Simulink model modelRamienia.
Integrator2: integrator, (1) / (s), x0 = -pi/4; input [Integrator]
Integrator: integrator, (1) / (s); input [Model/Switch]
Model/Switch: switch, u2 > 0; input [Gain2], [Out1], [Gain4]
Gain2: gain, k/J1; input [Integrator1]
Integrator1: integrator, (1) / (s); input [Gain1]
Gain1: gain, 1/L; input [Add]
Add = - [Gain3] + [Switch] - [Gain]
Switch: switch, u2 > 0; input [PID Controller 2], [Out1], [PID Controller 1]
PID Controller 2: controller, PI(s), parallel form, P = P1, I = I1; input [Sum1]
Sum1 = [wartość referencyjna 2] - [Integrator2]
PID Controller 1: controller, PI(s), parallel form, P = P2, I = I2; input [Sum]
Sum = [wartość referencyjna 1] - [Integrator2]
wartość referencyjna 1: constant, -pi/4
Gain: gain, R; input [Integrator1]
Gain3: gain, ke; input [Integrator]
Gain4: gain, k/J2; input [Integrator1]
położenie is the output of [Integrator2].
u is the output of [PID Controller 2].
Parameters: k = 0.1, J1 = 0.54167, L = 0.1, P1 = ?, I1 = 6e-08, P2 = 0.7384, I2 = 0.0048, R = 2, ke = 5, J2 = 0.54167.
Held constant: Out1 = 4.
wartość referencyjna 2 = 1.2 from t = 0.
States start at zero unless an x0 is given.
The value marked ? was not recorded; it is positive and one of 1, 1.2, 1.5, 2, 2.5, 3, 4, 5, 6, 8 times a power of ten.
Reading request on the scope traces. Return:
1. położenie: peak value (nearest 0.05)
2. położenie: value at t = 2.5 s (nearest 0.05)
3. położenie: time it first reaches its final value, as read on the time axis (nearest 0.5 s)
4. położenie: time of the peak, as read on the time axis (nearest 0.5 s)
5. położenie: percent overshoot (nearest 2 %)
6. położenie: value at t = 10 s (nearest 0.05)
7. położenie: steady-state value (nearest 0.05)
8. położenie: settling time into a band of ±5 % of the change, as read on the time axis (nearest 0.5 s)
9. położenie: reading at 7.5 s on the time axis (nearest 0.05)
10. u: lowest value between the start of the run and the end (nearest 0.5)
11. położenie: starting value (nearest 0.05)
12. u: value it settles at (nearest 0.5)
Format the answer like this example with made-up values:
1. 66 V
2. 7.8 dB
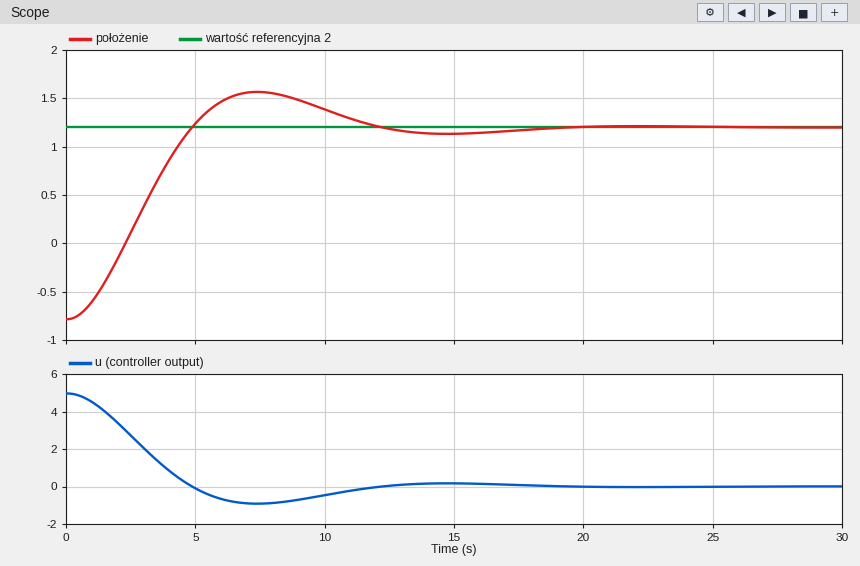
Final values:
1. 1.55
2. 0.10
3. 5.0 s
4. 7.5 s
5. 18 %
6. 1.40
7. 1.20
8. 11.0 s
9. 1.55
10. -1.0
11. -0.80
12. 0.0
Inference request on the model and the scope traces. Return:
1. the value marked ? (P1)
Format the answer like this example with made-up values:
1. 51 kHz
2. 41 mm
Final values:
1. 2.5
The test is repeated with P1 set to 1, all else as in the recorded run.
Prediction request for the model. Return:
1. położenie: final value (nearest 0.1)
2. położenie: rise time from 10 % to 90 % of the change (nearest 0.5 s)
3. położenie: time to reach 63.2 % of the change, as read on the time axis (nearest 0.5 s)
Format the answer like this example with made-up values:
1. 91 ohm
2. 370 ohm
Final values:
1. 1.2
2. 7.5 s
3. 6.0 s
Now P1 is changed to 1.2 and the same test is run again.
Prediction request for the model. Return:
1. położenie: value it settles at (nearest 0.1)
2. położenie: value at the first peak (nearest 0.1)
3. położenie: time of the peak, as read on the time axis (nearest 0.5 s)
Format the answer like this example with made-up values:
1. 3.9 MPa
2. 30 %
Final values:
1. 1.2
2. 1.3
3. 13.0 s
